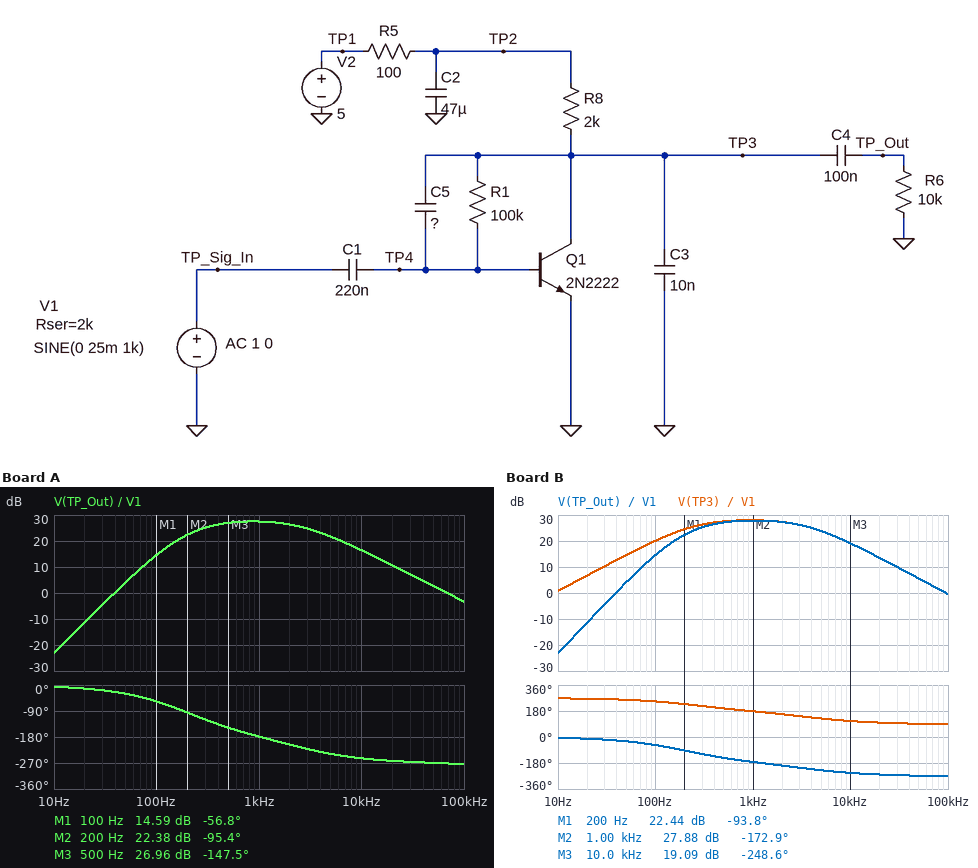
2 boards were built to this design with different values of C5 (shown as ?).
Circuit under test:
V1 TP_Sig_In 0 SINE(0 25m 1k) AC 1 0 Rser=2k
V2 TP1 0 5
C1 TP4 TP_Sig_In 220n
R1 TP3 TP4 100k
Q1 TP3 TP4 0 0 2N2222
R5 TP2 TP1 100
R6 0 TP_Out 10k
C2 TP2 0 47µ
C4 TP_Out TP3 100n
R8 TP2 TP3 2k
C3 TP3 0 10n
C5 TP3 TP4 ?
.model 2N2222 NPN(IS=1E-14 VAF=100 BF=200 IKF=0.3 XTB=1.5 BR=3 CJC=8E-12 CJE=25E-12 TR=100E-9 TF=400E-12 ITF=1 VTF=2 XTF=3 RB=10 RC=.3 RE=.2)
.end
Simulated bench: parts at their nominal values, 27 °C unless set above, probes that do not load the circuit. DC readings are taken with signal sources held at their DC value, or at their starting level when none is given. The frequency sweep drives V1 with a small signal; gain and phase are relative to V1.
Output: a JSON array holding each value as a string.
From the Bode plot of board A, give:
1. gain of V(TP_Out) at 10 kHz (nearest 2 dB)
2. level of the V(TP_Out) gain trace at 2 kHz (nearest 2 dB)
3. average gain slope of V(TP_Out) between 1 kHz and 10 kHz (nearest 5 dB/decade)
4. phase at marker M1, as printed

["16 dB", "26 dB", "-10 dB/decade", "-56.8 deg"]
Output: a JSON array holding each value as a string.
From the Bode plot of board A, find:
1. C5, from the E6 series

["1 nF"]
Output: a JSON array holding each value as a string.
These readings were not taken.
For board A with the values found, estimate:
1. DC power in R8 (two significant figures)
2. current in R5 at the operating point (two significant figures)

["5.6 mW", "1.7 mA"]
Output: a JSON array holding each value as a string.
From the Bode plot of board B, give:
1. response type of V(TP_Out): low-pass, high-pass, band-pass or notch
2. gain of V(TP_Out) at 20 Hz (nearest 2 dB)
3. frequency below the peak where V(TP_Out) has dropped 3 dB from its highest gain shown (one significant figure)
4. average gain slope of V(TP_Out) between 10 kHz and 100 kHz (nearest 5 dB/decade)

["band-pass", "-12 dB", "300 Hz", "-20 dB/decade"]
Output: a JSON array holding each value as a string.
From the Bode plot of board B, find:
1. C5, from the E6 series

["680 pF"]
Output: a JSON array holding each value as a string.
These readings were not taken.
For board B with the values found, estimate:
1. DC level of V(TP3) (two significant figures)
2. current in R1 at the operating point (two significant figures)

["1.5 V", "8.3 µA"]
